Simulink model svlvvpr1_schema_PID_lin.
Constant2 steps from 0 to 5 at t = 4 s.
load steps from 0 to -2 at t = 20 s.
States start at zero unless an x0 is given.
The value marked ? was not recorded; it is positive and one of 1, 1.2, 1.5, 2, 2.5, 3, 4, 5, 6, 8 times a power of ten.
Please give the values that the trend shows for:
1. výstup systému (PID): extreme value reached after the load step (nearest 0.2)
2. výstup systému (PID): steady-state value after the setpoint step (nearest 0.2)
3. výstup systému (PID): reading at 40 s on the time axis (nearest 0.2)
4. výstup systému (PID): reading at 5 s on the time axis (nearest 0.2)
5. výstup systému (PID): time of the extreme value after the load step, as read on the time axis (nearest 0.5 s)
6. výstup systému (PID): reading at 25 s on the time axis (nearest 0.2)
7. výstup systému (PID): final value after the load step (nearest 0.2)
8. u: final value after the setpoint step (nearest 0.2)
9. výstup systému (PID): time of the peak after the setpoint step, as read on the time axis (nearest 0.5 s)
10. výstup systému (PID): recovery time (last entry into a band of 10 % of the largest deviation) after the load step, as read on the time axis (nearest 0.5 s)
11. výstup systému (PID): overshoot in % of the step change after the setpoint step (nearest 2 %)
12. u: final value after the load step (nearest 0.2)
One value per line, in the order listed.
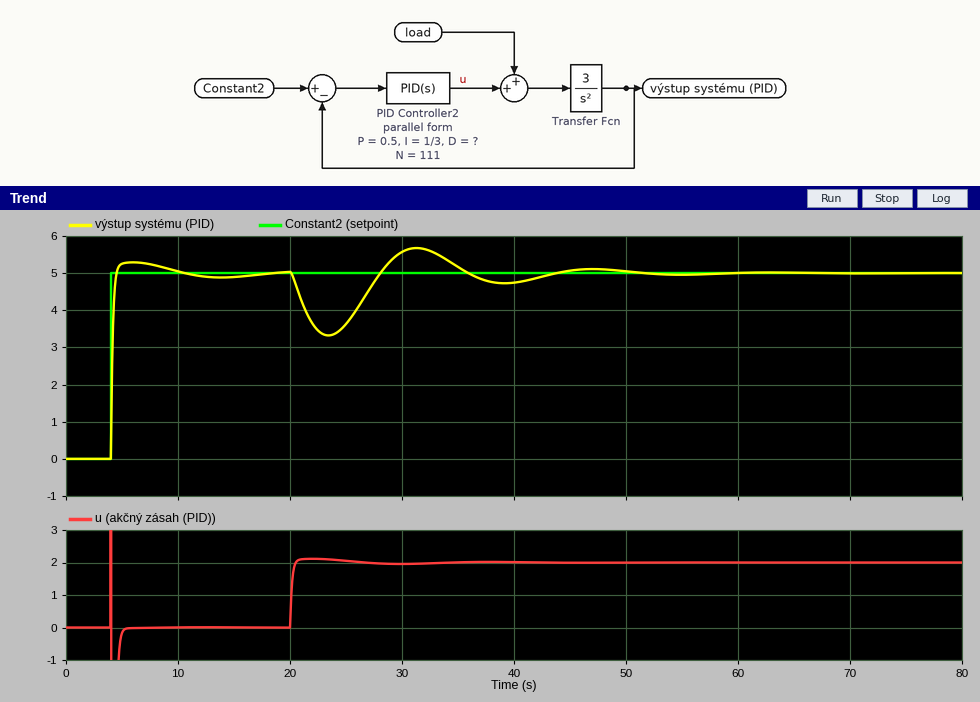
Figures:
3.4
5.0
4.8
5.2
23.5 s
3.6
5.0
0.0
6.0 s
41.5 s
6 %
2.0
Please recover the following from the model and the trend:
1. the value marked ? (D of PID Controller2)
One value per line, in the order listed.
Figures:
2
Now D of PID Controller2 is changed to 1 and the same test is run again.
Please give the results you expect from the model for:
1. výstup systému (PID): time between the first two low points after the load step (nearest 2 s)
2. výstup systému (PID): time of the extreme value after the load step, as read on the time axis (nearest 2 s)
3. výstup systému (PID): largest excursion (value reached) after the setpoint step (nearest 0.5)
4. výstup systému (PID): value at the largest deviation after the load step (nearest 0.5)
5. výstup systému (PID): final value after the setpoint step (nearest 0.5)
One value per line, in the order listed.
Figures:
10 s
22 s
6.0
2.5
5.0
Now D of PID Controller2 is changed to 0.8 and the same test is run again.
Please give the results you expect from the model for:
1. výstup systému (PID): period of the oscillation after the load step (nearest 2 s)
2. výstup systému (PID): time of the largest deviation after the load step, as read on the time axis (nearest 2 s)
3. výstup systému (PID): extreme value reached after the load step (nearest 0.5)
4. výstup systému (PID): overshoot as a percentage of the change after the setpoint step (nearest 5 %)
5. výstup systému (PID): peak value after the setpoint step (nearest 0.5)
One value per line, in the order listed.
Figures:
10 s
22 s
2.5
25 %
6.0
